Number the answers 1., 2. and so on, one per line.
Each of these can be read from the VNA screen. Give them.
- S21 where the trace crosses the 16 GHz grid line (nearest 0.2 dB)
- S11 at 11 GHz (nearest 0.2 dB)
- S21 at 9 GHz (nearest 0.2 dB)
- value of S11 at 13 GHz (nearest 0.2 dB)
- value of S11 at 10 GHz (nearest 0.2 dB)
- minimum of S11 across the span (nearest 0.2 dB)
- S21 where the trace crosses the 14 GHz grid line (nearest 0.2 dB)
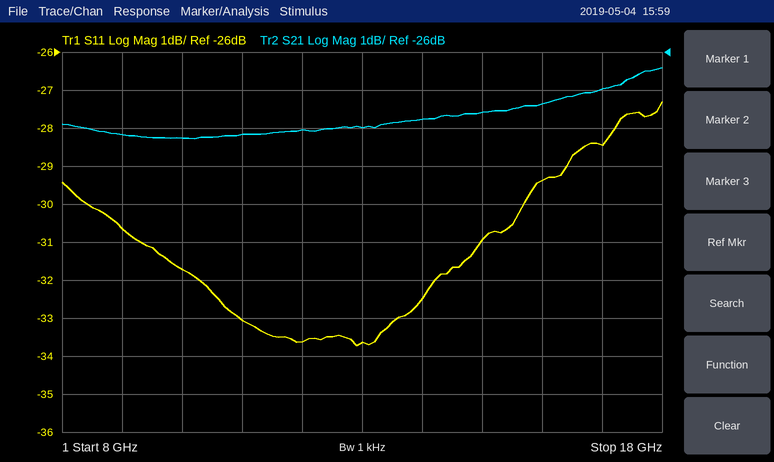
1. -27.4 dB
2. -33.0 dB
3. -28.2 dB
4. -33.6 dB
5. -31.8 dB
6. -33.8 dB
7. -27.8 dB
